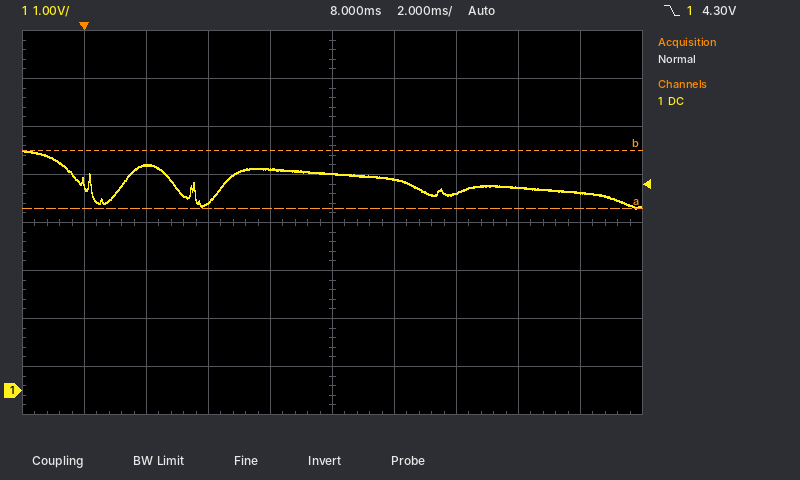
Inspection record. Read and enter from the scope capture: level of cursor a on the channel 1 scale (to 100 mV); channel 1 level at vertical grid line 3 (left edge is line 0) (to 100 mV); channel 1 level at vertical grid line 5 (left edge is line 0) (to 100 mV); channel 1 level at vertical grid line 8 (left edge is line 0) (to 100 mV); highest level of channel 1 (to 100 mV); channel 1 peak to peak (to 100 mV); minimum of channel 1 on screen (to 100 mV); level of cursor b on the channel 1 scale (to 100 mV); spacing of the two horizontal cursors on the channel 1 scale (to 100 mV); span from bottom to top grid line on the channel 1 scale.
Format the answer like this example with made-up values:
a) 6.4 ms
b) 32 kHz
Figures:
a) 3.8 V
b) 3.9 V
c) 4.5 V
d) 4.2 V
e) 5.0 V
f) 1.2 V
g) 3.8 V
h) 5.0 V
i) 1.2 V
j) 8 V
